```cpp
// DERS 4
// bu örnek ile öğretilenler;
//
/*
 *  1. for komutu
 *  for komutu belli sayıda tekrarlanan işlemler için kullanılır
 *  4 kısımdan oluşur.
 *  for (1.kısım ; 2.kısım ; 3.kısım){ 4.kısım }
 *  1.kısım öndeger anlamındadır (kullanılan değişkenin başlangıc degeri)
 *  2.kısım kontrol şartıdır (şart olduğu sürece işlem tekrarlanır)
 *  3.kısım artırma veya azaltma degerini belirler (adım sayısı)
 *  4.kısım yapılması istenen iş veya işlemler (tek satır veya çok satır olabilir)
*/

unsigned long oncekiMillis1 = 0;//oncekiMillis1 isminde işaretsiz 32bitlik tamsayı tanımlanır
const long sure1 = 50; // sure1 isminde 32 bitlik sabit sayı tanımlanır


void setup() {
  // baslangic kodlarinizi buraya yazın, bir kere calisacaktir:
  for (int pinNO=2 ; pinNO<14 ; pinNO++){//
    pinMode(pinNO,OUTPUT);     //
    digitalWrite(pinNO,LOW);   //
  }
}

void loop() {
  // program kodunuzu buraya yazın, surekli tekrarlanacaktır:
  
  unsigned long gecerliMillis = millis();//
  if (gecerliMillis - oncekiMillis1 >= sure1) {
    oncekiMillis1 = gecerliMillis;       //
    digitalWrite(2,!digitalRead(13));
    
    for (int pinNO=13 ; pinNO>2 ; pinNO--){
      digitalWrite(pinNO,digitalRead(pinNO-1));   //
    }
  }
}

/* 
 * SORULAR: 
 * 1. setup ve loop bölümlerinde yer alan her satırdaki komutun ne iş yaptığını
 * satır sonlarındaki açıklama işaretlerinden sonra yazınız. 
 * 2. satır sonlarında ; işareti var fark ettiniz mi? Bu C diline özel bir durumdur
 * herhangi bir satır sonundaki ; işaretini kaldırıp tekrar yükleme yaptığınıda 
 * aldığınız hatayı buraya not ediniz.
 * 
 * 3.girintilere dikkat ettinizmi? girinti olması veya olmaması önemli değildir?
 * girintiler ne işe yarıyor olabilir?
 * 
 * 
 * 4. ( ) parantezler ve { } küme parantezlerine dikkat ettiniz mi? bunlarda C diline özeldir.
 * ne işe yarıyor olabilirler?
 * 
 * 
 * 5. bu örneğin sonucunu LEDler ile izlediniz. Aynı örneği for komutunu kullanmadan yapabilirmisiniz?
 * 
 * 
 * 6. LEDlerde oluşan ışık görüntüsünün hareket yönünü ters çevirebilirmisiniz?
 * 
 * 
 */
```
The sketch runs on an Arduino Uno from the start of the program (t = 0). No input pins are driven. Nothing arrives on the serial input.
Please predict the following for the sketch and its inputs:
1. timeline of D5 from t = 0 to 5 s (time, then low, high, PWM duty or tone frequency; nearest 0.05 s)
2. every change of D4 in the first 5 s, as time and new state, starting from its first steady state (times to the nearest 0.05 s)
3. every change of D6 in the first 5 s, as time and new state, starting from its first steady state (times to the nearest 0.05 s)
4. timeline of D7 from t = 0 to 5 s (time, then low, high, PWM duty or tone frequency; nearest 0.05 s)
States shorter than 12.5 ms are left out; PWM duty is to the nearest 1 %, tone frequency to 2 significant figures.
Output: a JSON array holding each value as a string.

["0 s low; 0.15 s high; 0.7 s low; 1.25 s high; 1.8 s low; 2.35 s high; 2.9 s low; 3.45 s high; 4 s low; 4.55 s high", "0 s low; 0.1 s high; 0.65 s low; 1.2 s high; 1.75 s low; 2.3 s high; 2.85 s low; 3.4 s high; 3.95 s low; 4.5 s high", "0 s low; 0.2 s high; 0.75 s low; 1.3 s high; 1.85 s low; 2.4 s high; 2.95 s low; 3.5 s high; 4.05 s low; 4.6 s high", "0 s low; 0.25 s high; 0.8 s low; 1.35 s high; 1.9 s low; 2.45 s high; 3 s low; 3.55 s high; 4.1 s low; 4.65 s high"]
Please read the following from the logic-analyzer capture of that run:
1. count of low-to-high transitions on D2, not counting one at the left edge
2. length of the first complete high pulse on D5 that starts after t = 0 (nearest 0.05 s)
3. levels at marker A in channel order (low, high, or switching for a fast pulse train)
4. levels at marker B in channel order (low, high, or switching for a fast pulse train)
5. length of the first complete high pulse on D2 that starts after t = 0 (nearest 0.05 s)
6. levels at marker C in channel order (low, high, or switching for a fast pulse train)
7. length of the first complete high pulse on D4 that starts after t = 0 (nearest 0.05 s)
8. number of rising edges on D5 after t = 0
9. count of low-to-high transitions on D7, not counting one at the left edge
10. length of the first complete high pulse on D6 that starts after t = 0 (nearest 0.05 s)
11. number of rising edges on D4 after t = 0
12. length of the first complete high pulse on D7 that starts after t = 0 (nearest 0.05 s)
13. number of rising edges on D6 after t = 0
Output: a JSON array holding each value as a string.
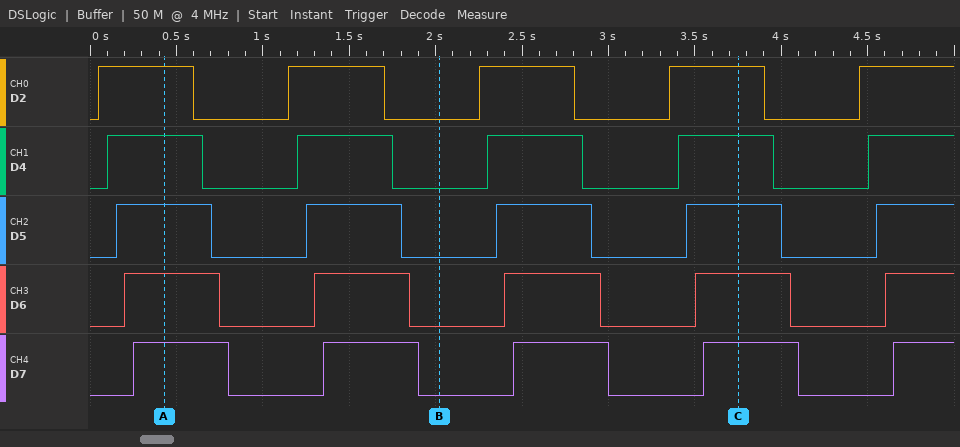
["5", "0.55 s", "D2 high, D4 high, D5 high, D6 high, D7 high", "D2 low, D4 low, D5 low, D6 low, D7 low", "0.55 s", "D2 high, D4 high, D5 high, D6 high, D7 high", "0.55 s", "5", "5", "0.55 s", "5", "0.55 s", "5"]
